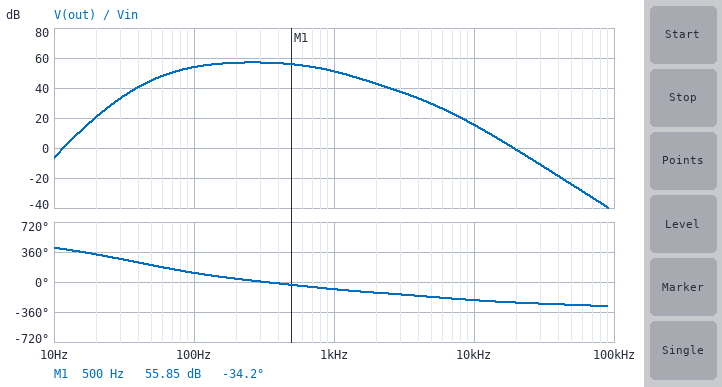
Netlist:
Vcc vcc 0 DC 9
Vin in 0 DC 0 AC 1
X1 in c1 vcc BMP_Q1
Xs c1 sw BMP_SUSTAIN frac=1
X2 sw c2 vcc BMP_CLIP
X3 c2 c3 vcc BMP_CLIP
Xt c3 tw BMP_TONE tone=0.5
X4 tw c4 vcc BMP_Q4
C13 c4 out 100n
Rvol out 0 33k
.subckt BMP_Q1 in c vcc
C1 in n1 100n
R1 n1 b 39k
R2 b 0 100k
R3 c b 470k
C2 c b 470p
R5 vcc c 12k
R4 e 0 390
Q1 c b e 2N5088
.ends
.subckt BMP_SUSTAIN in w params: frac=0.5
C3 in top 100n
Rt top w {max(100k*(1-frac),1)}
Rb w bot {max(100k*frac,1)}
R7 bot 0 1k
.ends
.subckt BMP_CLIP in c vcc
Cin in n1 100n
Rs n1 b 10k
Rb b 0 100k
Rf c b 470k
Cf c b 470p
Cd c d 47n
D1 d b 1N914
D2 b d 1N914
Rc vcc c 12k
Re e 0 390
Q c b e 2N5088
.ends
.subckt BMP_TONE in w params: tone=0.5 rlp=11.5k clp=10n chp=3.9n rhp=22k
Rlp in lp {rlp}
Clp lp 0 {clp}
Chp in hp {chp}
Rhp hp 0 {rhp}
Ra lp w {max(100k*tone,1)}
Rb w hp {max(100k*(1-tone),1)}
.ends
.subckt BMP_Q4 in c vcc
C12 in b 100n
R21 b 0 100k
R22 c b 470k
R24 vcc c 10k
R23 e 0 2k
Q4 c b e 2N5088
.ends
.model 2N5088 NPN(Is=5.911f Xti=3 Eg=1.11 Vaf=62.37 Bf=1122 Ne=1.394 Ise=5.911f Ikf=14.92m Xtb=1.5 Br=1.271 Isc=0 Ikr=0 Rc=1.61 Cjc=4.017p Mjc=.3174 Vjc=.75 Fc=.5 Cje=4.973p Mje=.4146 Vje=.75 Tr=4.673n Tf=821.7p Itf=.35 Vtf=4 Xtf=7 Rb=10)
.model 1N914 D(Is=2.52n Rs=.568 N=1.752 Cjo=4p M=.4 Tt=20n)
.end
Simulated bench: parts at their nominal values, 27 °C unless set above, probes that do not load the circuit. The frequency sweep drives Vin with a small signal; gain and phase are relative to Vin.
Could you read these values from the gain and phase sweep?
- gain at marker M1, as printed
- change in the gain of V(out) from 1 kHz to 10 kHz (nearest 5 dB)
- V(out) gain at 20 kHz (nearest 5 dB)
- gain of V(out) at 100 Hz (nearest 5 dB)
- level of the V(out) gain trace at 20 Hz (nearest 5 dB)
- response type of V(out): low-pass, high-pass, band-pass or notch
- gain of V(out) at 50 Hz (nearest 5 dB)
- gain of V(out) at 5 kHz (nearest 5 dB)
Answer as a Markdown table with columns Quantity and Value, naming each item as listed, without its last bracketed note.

| Quantity | Value |
|---|---|
| gain at marker M1, as printed | 55.85 dB |
| change in the gain of V(out) from 1 kHz to 10 kHz | -35 dB |
| V(out) gain at 20 kHz | 0 dB |
| gain of V(out) at 100 Hz | 55 dB |
| level of the V(out) gain trace at 20 Hz | 20 dB |
| response type of V(out): low-pass, high-pass, band-pass or notch | band-pass |
| gain of V(out) at 50 Hz | 45 dB |
| gain of V(out) at 5 kHz | 30 dB |
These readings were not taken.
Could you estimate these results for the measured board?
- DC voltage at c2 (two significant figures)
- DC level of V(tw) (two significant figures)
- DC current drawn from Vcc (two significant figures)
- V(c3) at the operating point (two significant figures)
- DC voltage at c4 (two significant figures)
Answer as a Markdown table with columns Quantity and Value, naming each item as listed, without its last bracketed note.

| Quantity | Value |
|---|---|
| DC voltage at c2 | 4.7 V |
| DC level of V(tw) | 2.5 V |
| DC current drawn from Vcc | 1.3 mA |
| V(c3) at the operating point | 4.6 V |
| DC voltage at c4 | 6.5 V |
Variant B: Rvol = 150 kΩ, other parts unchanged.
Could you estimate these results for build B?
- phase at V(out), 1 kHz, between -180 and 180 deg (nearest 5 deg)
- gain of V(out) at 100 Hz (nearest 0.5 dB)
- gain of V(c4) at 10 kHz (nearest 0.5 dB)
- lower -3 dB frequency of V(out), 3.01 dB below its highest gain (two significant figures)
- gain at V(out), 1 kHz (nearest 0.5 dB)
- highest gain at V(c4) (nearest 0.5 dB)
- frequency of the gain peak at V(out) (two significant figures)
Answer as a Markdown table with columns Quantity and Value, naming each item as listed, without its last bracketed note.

| Quantity | Value |
|---|---|
| phase at V(out), 1 kHz, between -180 and 180 deg | -90 deg |
| gain of V(out) at 100 Hz | 56.0 dB |
| gain of V(c4) at 10 kHz | 17.0 dB |
| lower -3 dB frequency of V(out), 3.01 dB below its highest gain | 95 Hz |
| gain at V(out), 1 kHz | 52.5 dB |
| highest gain at V(c4) | 58.5 dB |
| frequency of the gain peak at V(out) | 250 Hz |
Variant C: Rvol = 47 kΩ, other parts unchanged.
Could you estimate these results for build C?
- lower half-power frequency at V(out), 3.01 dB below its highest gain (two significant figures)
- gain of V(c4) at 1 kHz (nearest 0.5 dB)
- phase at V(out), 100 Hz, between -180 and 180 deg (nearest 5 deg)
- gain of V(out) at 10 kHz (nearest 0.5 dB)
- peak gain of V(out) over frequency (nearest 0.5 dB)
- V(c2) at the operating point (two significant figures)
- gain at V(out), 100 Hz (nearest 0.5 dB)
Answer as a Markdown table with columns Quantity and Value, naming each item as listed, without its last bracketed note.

| Quantity | Value |
|---|---|
| lower half-power frequency at V(out), 3.01 dB below its highest gain | 99 Hz |
| gain of V(c4) at 1 kHz | 51.5 dB |
| phase at V(out), 100 Hz, between -180 and 180 deg | 105 deg |
| gain of V(out) at 10 kHz | 16.0 dB |
| peak gain of V(out) over frequency | 57.5 dB |
| V(c2) at the operating point | 4.7 V |
| gain at V(out), 100 Hz | 54.5 dB |
